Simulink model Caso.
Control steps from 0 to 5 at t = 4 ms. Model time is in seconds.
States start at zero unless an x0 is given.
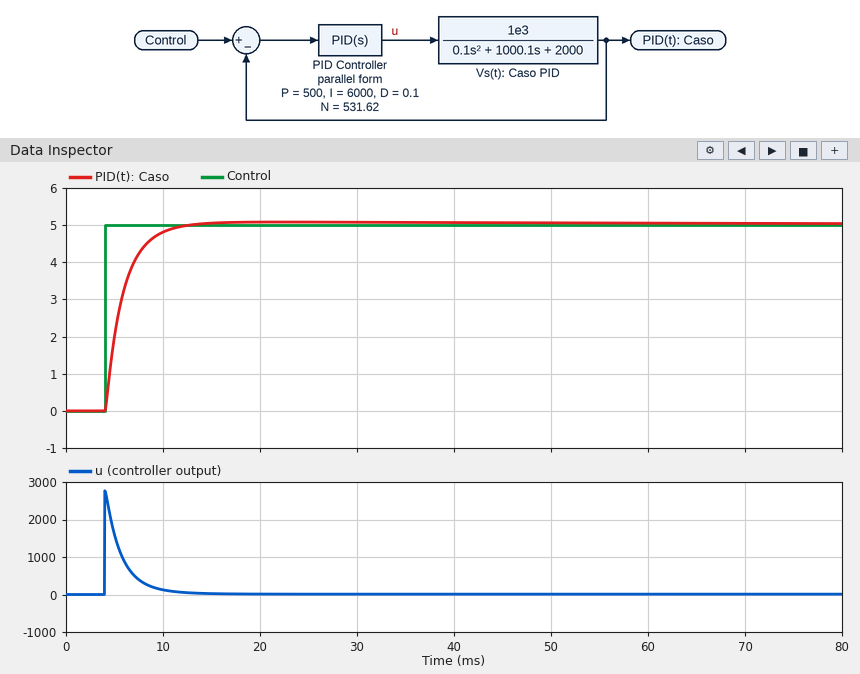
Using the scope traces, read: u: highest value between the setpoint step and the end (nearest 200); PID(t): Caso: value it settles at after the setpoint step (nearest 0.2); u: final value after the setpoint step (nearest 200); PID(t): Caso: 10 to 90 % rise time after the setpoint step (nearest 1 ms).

2800
5.0
0
4 ms
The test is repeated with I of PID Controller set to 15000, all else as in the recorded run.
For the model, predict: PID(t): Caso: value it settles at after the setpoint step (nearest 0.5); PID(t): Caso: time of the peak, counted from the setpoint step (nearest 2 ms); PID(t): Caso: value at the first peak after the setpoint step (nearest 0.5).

5.0
14 ms
5.0
